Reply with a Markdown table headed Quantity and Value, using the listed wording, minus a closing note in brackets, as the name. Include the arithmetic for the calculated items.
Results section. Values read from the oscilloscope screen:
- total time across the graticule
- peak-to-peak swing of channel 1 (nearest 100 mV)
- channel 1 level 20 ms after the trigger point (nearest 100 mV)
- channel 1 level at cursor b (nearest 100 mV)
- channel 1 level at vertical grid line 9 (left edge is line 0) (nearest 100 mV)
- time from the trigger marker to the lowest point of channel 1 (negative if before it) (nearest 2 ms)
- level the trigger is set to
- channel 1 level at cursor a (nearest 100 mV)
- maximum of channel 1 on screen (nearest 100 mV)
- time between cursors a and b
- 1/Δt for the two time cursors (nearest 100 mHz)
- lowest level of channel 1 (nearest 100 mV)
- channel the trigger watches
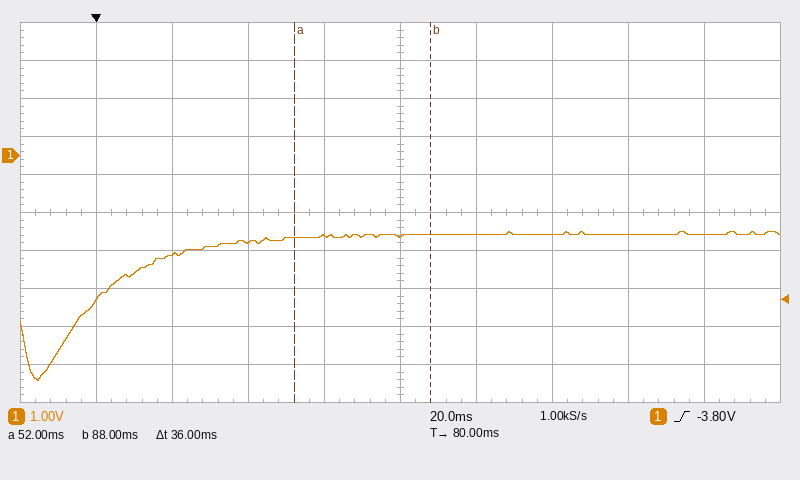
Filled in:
| Quantity | Value |
|---|---|
| total time across the graticule | 200 ms |
| peak-to-peak swing of channel 1 | -2.0 V − (-5.9 V) = 3.9 V |
| channel 1 level 20 ms after the trigger point | -2.6 V |
| channel 1 level at cursor b | -2.1 V |
| channel 1 level at vertical grid line 9 (left edge is line 0) | -2.1 V |
| time from the trigger marker to the lowest point of channel 1 (negative if before it) | -16 ms |
| level the trigger is set to | -3.80 V |
| channel 1 level at cursor a | -2.2 V |
| maximum of channel 1 on screen | -2.0 V |
| time between cursors a and b | 36 ms |
| 1/Δt for the two time cursors | 1 / 36 ms ≈ 27.8 Hz |
| lowest level of channel 1 | -5.9 V |
| channel the trigger watches | channel 1 |
